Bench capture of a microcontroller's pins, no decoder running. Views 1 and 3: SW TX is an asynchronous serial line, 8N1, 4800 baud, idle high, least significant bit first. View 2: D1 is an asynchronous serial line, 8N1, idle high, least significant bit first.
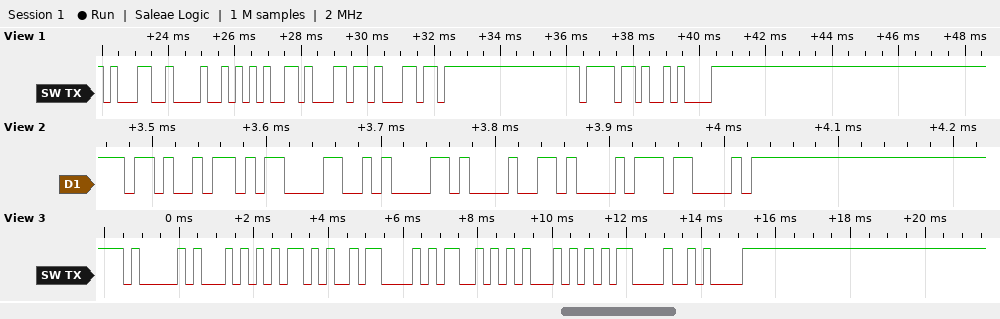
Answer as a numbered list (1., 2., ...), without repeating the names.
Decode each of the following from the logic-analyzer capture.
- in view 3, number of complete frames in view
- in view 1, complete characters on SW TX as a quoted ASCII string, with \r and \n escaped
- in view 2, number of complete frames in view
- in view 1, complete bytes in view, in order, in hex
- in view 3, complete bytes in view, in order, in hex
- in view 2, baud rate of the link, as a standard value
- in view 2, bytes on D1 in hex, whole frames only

1. 8
2. "1Hello\n"
3. 6
4. 31 48 65 6C 6C 6F 0A
5. 0x41 0x54 0x2B 0x43 0x53 0x51 0x0D 0x0A
6. 115200 baud
7. 4B 0D 0A 21 A1 43
